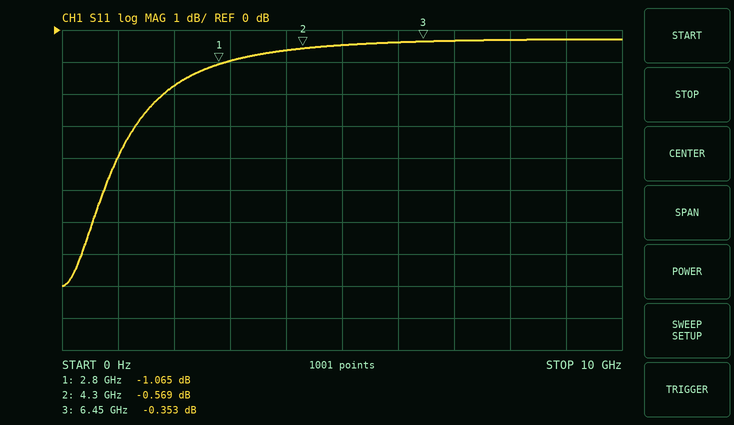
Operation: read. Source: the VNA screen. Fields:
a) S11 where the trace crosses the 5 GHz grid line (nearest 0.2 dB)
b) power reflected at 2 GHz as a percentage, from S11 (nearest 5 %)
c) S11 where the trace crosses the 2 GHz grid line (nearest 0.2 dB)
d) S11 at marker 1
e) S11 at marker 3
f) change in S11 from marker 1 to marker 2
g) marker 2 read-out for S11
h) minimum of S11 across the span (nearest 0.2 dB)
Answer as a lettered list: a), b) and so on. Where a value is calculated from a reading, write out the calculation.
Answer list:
a) -0.4 dB
b) 10^(-1.8/10) ≈ 66.1 %, so 65 % to the nearest 5 %
c) -1.8 dB
d) -1.065 dB
e) -0.353 dB
f) -0.569 − (-1.065) = 0.496 dB
g) -0.569 dB
h) -8.0 dB
